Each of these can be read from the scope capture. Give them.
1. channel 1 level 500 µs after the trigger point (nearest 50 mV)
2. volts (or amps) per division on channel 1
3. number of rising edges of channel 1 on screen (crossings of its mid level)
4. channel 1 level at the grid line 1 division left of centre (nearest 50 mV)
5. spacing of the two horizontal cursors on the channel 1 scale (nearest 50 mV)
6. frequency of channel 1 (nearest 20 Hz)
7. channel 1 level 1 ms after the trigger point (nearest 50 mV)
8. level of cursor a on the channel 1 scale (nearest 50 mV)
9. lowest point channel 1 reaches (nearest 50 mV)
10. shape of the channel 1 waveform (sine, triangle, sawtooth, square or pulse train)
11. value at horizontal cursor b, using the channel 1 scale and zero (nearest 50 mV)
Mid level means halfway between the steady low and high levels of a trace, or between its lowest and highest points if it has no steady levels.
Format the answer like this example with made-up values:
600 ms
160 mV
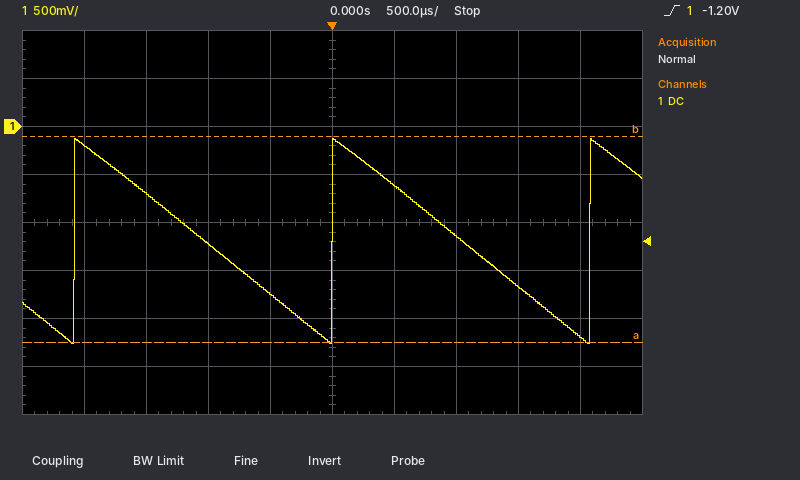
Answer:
-600 mV
500 mV
3
-1.75 V
2.15 V
480 Hz
-1.15 V
-2.25 V
-2.25 V
sawtooth
-100 mV
